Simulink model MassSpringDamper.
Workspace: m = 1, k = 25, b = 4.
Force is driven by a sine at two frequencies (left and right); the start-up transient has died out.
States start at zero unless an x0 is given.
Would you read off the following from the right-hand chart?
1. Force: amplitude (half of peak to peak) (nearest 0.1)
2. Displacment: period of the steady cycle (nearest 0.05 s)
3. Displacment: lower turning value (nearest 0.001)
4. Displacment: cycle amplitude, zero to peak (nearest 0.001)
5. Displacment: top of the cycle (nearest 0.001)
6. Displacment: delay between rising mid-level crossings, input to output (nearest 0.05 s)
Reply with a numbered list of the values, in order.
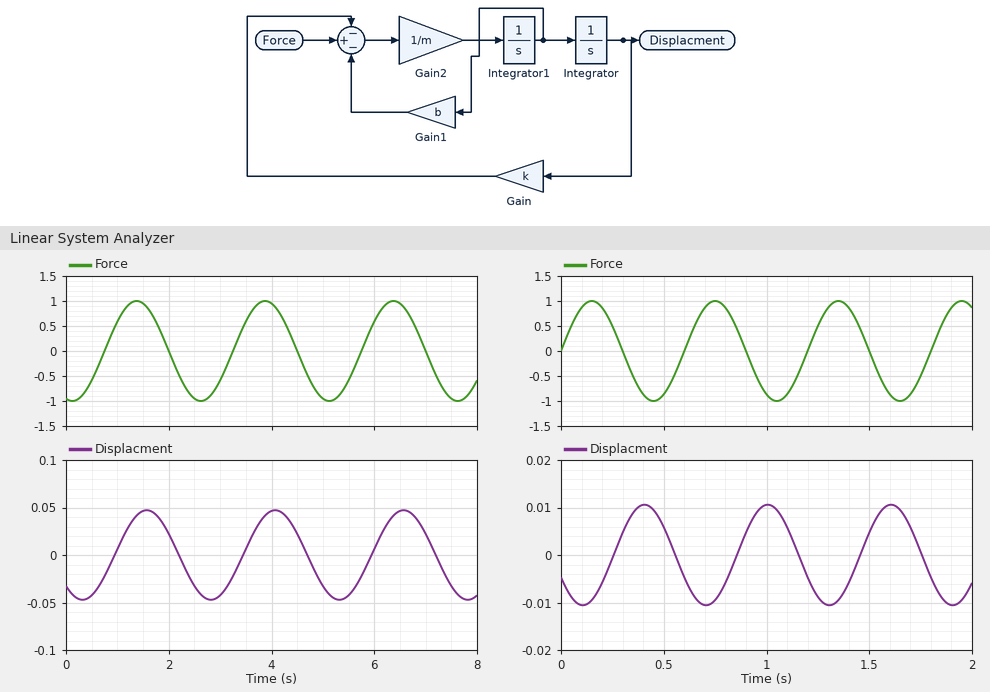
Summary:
1. 1.0
2. 0.60 s
3. -0.011
4. 0.011
5. 0.011
6. 0.25 s
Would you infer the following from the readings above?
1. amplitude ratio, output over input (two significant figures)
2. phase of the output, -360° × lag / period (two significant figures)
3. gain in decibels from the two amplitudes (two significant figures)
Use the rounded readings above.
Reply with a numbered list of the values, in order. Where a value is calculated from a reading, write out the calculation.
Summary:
1. 0.011 / 1 = 0.011
2. -360 × 0.25 / 0.6 = -150°
3. 20 log10(0.011 / 1) = -39 dB
